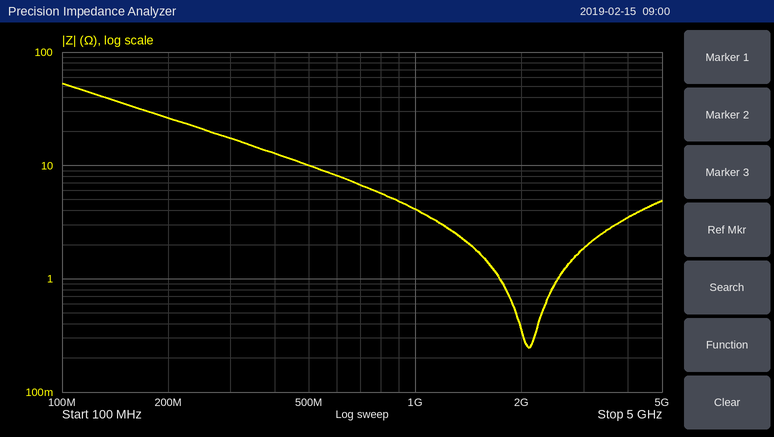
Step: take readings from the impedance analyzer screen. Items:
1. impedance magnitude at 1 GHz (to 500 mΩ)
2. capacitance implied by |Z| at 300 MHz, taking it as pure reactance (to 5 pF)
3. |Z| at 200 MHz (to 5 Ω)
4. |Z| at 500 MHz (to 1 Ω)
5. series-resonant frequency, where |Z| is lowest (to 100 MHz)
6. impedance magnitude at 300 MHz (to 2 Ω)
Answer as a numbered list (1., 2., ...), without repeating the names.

1. 4.0 Ω
2. 30 pF
3. 25 Ω
4. 10 Ω
5. 2.1 GHz
6. 18 Ω
